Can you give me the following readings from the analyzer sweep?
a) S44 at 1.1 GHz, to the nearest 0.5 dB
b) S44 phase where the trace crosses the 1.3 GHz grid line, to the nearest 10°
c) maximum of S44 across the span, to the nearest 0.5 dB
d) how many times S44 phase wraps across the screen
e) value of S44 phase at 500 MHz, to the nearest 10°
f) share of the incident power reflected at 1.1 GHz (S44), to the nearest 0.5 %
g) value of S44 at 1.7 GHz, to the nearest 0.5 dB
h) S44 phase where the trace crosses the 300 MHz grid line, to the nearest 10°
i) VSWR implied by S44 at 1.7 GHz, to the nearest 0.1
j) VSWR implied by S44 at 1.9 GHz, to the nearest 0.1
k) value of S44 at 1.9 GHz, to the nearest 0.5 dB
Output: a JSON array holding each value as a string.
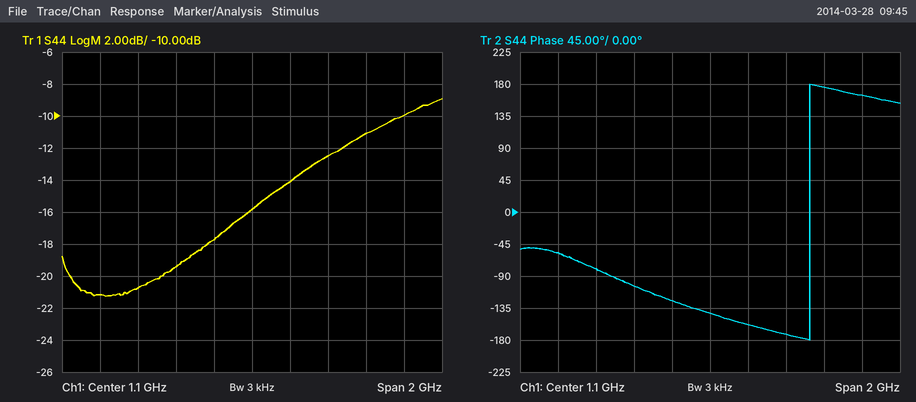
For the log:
["-16.0 dB", "-160°", "-9.0 dB", "1", "-80°", "2.5 %", "-11.0 dB", "-60°", "1.8", "1.9", "-10.0 dB"]
